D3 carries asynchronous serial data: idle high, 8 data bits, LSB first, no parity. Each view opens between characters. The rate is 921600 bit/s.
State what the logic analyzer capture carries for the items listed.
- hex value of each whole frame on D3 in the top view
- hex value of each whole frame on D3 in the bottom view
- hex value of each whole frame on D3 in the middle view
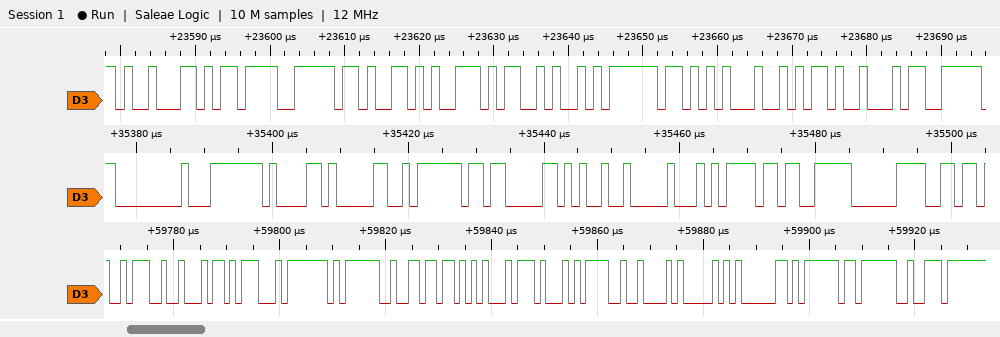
89, ED, BE, 59, AE, 4A, BF, 15, 6A, A2
3A, A2, 1D, 7F, 3F, B6, 15, 17, 3D, 42, 50, 60, BF, 3F, EE
00, FC, 61, 30, BF, 83, 25, 10, BD, F3, E0
